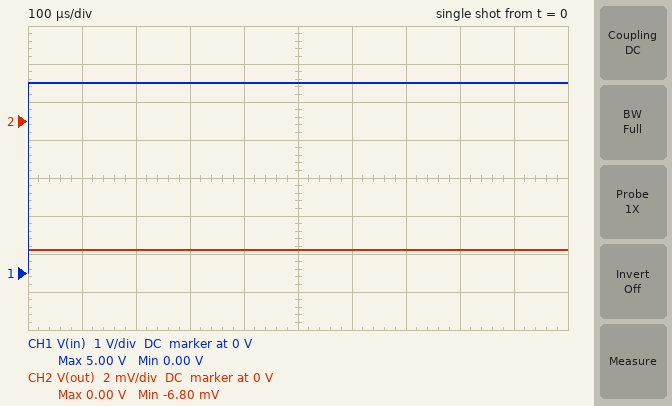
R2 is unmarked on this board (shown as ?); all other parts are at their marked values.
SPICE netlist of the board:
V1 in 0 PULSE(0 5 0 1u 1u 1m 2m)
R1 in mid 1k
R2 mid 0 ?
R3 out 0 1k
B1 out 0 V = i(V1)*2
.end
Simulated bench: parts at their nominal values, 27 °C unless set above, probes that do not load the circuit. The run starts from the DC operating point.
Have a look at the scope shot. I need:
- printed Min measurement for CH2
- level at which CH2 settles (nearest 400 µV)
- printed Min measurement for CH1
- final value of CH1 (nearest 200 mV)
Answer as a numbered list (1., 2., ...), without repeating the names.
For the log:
1. -6.80 mV
2. -6.8 mV
3. 0.00 V
4. 5.0 V
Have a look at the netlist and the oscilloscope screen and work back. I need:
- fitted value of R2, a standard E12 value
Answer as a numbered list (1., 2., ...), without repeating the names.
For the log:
1. 470 Ω
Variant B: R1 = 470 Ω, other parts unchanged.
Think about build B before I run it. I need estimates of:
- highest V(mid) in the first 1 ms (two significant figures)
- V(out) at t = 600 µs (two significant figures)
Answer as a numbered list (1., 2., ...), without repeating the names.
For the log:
1. 2.5 V
2. -11 mV
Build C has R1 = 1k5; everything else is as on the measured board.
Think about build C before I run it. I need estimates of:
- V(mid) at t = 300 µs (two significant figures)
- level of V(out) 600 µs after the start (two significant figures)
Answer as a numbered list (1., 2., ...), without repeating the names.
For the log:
1. 1.2 V
2. -5.1 mV
